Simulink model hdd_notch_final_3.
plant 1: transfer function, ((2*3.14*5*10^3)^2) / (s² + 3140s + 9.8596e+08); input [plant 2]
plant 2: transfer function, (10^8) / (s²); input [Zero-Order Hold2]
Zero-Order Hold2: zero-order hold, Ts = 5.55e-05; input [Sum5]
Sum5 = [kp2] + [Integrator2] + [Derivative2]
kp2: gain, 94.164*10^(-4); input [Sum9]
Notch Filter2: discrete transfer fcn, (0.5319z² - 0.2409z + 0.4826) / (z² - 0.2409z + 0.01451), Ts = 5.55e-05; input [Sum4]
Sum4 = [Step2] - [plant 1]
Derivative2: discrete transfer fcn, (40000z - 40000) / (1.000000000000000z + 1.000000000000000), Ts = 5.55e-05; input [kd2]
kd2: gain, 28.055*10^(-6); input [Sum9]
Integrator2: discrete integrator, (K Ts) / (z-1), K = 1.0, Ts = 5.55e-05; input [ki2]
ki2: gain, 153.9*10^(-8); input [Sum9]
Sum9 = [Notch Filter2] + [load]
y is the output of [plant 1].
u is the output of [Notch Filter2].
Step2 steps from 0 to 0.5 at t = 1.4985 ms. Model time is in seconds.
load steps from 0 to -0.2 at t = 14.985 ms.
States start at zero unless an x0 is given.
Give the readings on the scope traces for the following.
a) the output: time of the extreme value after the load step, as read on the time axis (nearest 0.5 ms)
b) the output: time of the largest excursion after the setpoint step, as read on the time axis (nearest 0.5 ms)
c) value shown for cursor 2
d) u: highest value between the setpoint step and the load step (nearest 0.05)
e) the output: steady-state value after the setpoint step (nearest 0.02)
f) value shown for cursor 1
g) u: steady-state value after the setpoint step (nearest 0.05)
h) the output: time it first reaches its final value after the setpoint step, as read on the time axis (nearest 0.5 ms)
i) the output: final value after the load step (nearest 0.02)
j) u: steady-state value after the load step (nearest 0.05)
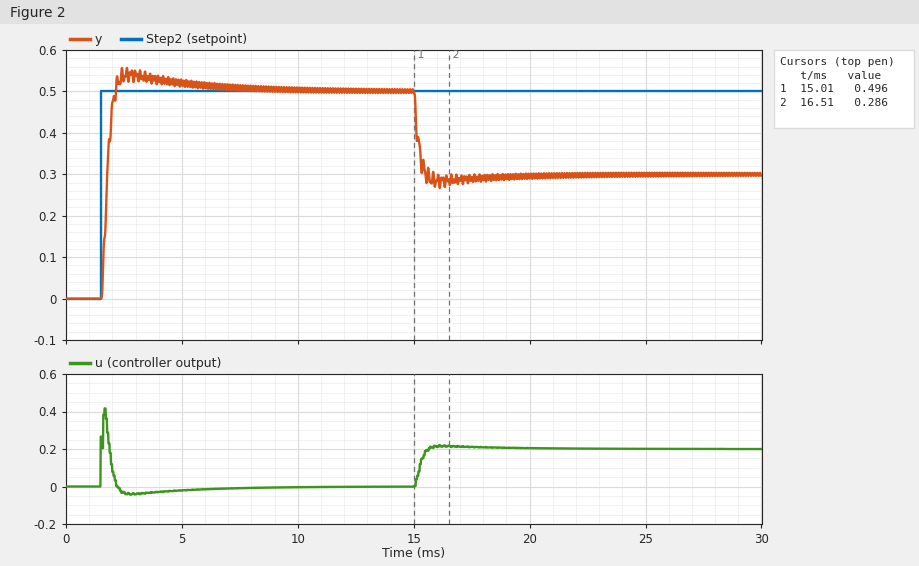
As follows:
16.0 ms
2.5 ms
0.286
0.40
0.50
0.496
0.00
2.0 ms
0.30
0.20
